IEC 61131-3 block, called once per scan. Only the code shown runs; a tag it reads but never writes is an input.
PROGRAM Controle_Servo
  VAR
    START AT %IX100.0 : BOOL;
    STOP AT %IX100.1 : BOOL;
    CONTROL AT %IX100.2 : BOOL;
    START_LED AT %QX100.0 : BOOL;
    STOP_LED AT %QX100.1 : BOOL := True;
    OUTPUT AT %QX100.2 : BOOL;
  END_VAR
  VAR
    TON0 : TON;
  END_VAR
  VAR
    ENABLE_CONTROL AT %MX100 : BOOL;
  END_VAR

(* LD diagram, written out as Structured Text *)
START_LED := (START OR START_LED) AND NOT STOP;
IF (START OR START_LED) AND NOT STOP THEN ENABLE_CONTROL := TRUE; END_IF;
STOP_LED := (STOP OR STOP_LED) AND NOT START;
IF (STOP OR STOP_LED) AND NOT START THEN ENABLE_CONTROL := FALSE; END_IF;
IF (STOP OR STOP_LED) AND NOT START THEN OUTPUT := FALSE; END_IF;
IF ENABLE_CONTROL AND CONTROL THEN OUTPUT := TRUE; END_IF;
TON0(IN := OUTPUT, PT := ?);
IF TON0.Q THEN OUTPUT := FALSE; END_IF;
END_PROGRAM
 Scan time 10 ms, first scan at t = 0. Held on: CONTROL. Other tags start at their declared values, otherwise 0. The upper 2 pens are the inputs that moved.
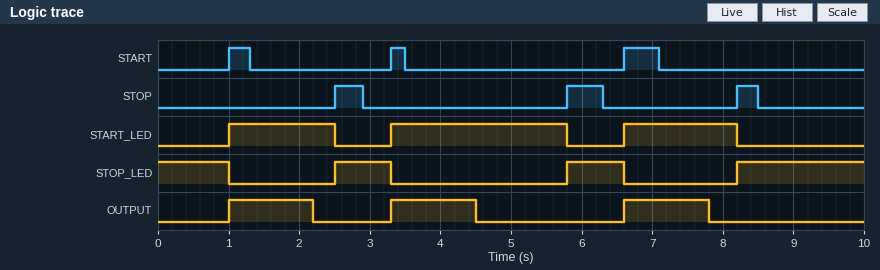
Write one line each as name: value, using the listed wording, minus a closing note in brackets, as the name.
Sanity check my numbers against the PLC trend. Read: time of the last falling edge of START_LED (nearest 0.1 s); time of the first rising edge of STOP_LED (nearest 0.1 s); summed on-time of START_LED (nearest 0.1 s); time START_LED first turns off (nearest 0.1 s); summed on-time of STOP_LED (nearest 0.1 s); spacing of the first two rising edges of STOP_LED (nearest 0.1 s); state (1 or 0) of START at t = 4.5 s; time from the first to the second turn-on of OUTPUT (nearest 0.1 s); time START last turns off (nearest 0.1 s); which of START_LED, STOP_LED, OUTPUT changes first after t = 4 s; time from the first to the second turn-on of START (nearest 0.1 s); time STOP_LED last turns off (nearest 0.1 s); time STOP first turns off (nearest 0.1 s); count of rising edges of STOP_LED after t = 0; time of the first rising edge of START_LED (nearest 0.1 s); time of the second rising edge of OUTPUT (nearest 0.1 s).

time of the last falling edge of START_LED: 8.2 s
time of the first rising edge of STOP_LED: 2.5 s
summed on-time of START_LED: 5.6 s
time START_LED first turns off: 2.5 s
summed on-time of STOP_LED: 4.4 s
spacing of the first two rising edges of STOP_LED: 3.3 s
state (1 or 0) of START at t = 4.5 s: 0
time from the first to the second turn-on of OUTPUT: 2.3 s
time START last turns off: 7.1 s
which of START_LED, STOP_LED, OUTPUT changes first after t = 4 s: OUTPUT
time from the first to the second turn-on of START: 2.3 s
time STOP_LED last turns off: 6.6 s
time STOP first turns off: 2.9 s
count of rising edges of STOP_LED after t = 0: 3
time of the first rising edge of START_LED: 1.0 s
time of the second rising edge of OUTPUT: 3.3 s
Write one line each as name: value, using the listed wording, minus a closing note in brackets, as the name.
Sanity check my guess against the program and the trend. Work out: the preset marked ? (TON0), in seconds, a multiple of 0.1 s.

the preset marked ? (TON0), in seconds, a multiple of 0.1 s: 1.2 s
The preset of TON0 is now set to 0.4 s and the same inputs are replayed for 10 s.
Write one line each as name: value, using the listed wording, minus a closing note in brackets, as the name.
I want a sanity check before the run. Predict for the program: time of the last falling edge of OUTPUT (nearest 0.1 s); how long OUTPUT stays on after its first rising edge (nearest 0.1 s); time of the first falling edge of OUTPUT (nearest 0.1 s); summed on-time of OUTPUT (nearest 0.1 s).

time of the last falling edge of OUTPUT: 7.0 s
how long OUTPUT stays on after its first rising edge: 0.4 s
time of the first falling edge of OUTPUT: 1.4 s
summed on-time of OUTPUT: 1.2 s
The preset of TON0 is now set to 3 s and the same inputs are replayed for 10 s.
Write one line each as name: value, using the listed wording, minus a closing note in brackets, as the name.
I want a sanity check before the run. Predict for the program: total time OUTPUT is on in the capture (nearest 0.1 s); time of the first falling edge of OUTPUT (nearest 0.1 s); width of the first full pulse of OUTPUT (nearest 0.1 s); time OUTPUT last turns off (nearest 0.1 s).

total time OUTPUT is on in the capture: 5.6 s
time of the first falling edge of OUTPUT: 2.5 s
width of the first full pulse of OUTPUT: 1.5 s
time OUTPUT last turns off: 8.2 s
